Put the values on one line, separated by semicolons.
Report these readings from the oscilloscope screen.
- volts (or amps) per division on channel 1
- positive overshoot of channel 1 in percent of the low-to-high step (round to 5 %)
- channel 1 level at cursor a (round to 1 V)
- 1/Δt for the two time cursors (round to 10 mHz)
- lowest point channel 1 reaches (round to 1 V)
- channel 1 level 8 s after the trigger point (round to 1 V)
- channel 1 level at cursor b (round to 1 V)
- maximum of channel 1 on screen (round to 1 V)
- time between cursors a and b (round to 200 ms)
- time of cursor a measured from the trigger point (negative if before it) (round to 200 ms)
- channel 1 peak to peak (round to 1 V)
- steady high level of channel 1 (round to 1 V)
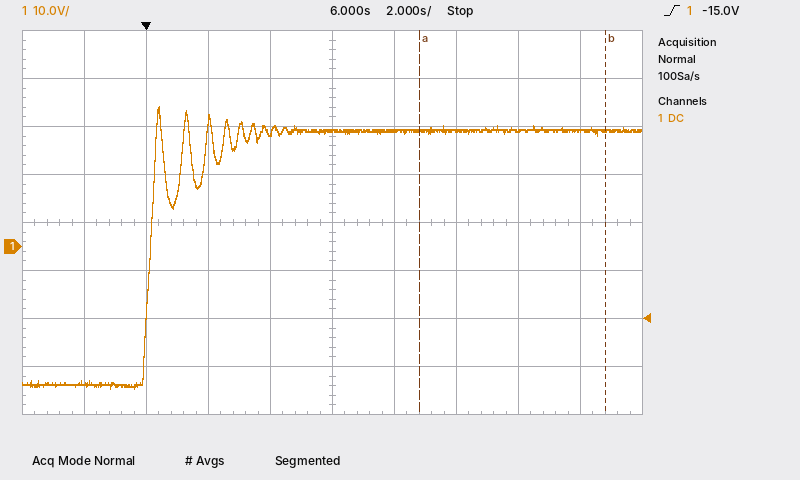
10 V; 10 %; 24 V; 170 mHz; -30 V; 24 V; 24 V; 29 V; 6.0 s; +8.8 s; 59 V; 24 V
